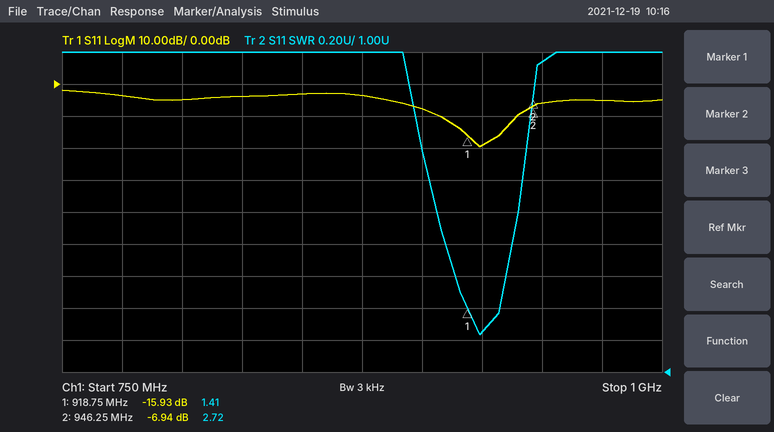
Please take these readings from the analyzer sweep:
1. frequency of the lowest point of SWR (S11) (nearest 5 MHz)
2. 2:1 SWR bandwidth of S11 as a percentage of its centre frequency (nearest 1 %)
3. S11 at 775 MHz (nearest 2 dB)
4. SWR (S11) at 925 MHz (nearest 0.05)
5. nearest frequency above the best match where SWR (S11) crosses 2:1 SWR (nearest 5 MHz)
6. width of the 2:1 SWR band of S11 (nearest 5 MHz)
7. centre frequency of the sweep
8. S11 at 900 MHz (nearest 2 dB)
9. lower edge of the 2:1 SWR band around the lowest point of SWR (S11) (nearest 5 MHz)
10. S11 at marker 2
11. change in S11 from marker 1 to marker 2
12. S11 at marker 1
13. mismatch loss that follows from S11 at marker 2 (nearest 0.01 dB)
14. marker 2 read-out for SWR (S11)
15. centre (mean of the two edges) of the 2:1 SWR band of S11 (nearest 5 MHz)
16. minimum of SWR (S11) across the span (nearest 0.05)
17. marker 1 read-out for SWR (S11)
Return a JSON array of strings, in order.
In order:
["925 MHz", "4 %", "-4 dB", "1.25", "940 MHz", "35 MHz", "875 MHz", "-8 dB", "905 MHz", "-6.94 dB", "8.99 dB", "-15.93 dB", "0.98 dB", "2.72", "925 MHz", "1.25", "1.41"]
